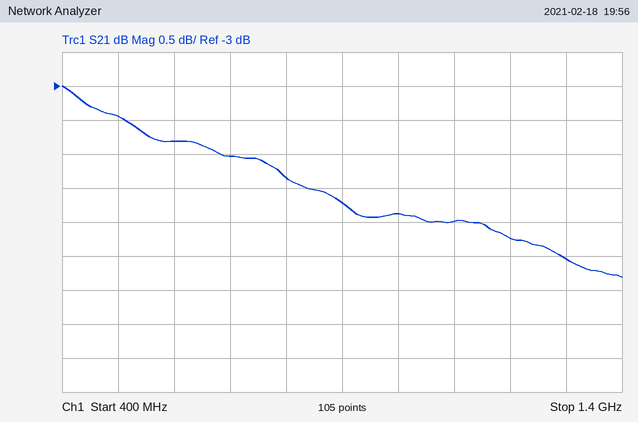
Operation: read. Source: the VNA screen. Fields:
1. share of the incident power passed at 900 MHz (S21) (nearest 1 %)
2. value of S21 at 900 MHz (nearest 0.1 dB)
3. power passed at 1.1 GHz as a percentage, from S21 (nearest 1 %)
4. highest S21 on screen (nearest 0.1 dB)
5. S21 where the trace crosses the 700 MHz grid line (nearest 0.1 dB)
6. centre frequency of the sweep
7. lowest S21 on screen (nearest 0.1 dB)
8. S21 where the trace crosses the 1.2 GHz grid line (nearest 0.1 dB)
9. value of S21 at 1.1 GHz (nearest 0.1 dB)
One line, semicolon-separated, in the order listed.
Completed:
34 %; -4.7 dB; 32 %; -3.0 dB; -4.0 dB; 900 MHz; -5.8 dB; -5.2 dB; -5.0 dB
